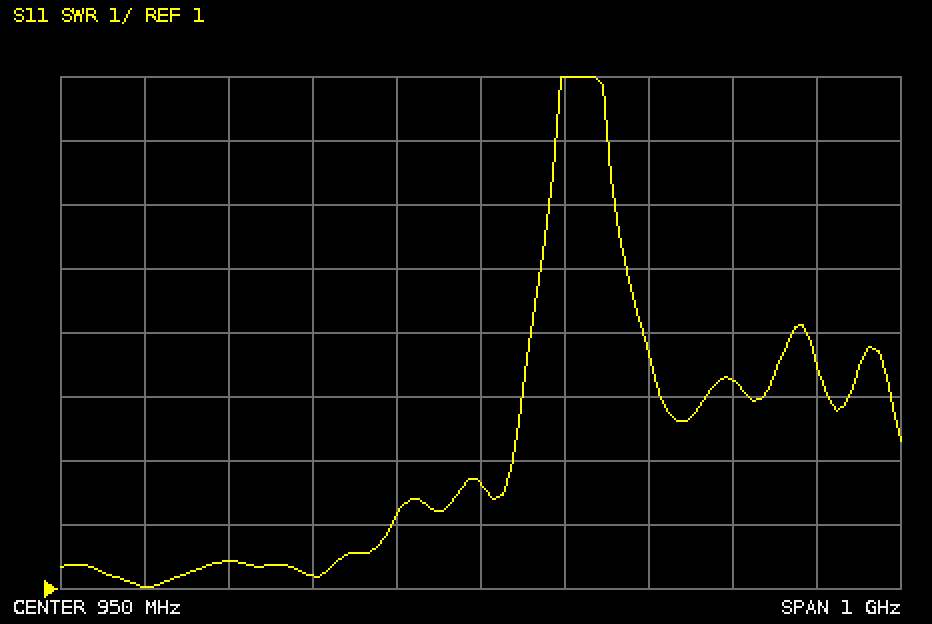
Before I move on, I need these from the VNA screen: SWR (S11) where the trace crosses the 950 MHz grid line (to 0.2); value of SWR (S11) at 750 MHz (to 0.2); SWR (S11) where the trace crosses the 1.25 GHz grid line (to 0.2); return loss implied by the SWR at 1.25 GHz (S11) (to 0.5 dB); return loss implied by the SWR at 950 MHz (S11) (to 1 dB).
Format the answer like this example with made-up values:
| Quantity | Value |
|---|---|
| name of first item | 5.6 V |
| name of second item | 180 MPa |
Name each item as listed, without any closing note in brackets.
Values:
| Quantity | Value |
|---|---|
| SWR (S11) where the trace crosses the 950 MHz grid line | 2.6 |
| value of SWR (S11) at 750 MHz | 1.2 |
| SWR (S11) where the trace crosses the 1.25 GHz grid line | 4.2 |
| return loss implied by the SWR at 1.25 GHz (S11) | 4.0 dB |
| return loss implied by the SWR at 950 MHz (S11) | 7 dB |
